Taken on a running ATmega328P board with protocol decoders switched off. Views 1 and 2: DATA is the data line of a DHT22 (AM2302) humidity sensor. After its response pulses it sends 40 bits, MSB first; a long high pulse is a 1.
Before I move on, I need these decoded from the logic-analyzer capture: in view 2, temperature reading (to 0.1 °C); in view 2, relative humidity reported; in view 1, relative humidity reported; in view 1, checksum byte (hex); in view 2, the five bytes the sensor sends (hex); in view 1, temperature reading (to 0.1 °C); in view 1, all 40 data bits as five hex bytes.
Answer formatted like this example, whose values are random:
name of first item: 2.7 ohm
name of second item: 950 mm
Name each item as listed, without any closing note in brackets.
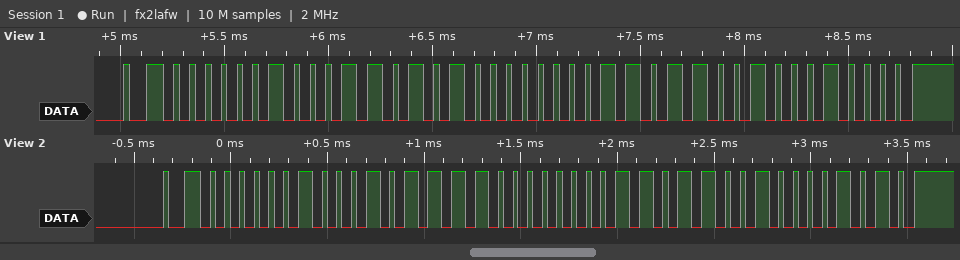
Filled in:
in view 2, temperature reading: 21.7 °C
in view 2, relative humidity reported: 55.9 %
in view 1, relative humidity reported: 56.5 %
in view 1, checksum byte: 0x10
in view 2, the five bytes the sensor sends: 02 2F 00 D9 0A
in view 1, temperature reading: 21.7 °C
in view 1, all 40 data bits as five hex bytes: 02 35 00 D9 10
